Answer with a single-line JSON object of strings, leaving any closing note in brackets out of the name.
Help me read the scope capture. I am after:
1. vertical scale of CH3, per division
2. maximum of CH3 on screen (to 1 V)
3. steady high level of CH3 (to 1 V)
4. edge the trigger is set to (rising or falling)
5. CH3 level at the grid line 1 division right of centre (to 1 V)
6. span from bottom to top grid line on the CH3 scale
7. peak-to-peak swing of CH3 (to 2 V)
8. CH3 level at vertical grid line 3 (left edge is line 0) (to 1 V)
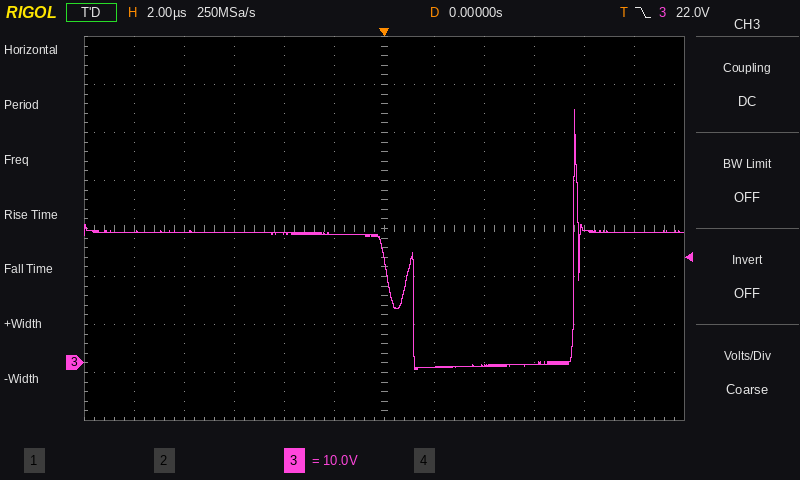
{"vertical scale of CH3, per division": "10 V", "maximum of CH3 on screen": "53 V", "steady high level of CH3": "27 V", "edge the trigger is set to": "falling", "CH3 level at the grid line 1 division right of centre": "-1 V", "span from bottom to top grid line on the CH3 scale": "80 V", "peak-to-peak swing of CH3": "54 V", "CH3 level at vertical grid line 3 (left edge is line 0)": "27 V"}
